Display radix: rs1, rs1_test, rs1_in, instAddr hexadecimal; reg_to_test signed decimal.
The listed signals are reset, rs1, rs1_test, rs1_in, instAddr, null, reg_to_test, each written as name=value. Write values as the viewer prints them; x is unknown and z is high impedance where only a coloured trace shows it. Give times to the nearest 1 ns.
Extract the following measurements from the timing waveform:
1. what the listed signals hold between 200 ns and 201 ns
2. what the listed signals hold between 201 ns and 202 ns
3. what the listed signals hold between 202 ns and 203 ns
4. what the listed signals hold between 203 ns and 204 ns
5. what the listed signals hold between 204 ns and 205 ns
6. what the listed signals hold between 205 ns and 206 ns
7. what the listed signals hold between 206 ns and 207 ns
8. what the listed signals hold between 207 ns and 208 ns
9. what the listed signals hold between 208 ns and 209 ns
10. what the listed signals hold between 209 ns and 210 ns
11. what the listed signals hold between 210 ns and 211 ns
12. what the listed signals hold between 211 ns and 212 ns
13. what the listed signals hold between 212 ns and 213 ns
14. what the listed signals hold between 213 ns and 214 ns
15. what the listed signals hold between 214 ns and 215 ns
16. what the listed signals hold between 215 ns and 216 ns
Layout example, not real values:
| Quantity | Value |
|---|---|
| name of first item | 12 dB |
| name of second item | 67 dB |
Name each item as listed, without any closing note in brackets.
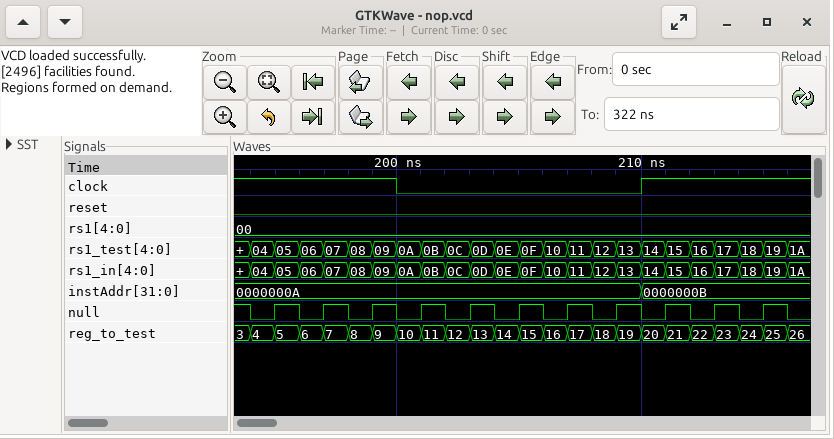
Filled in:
| Quantity | Value |
|---|---|
| what the listed signals hold between 200 ns and 201 ns | reset=0, rs1=00, rs1_test=0A, rs1_in=0A, instAddr=0000000A, null=0, reg_to_test=10 |
| what the listed signals hold between 201 ns and 202 ns | reset=0, rs1=00, rs1_test=0B, rs1_in=0B, instAddr=0000000A, null=1, reg_to_test=11 |
| what the listed signals hold between 202 ns and 203 ns | reset=0, rs1=00, rs1_test=0C, rs1_in=0C, instAddr=0000000A, null=0, reg_to_test=12 |
| what the listed signals hold between 203 ns and 204 ns | reset=0, rs1=00, rs1_test=0D, rs1_in=0D, instAddr=0000000A, null=1, reg_to_test=13 |
| what the listed signals hold between 204 ns and 205 ns | reset=0, rs1=00, rs1_test=0E, rs1_in=0E, instAddr=0000000A, null=0, reg_to_test=14 |
| what the listed signals hold between 205 ns and 206 ns | reset=0, rs1=00, rs1_test=0F, rs1_in=0F, instAddr=0000000A, null=1, reg_to_test=15 |
| what the listed signals hold between 206 ns and 207 ns | reset=0, rs1=00, rs1_test=10, rs1_in=10, instAddr=0000000A, null=0, reg_to_test=16 |
| what the listed signals hold between 207 ns and 208 ns | reset=0, rs1=00, rs1_test=11, rs1_in=11, instAddr=0000000A, null=1, reg_to_test=17 |
| what the listed signals hold between 208 ns and 209 ns | reset=0, rs1=00, rs1_test=12, rs1_in=12, instAddr=0000000A, null=0, reg_to_test=18 |
| what the listed signals hold between 209 ns and 210 ns | reset=0, rs1=00, rs1_test=13, rs1_in=13, instAddr=0000000A, null=1, reg_to_test=19 |
| what the listed signals hold between 210 ns and 211 ns | reset=0, rs1=00, rs1_test=14, rs1_in=14, instAddr=0000000B, null=0, reg_to_test=20 |
| what the listed signals hold between 211 ns and 212 ns | reset=0, rs1=00, rs1_test=15, rs1_in=15, instAddr=0000000B, null=1, reg_to_test=21 |
| what the listed signals hold between 212 ns and 213 ns | reset=0, rs1=00, rs1_test=16, rs1_in=16, instAddr=0000000B, null=0, reg_to_test=22 |
| what the listed signals hold between 213 ns and 214 ns | reset=0, rs1=00, rs1_test=17, rs1_in=17, instAddr=0000000B, null=1, reg_to_test=23 |
| what the listed signals hold between 214 ns and 215 ns | reset=0, rs1=00, rs1_test=18, rs1_in=18, instAddr=0000000B, null=0, reg_to_test=24 |
| what the listed signals hold between 215 ns and 216 ns | reset=0, rs1=00, rs1_test=19, rs1_in=19, instAddr=0000000B, null=1, reg_to_test=25 |
